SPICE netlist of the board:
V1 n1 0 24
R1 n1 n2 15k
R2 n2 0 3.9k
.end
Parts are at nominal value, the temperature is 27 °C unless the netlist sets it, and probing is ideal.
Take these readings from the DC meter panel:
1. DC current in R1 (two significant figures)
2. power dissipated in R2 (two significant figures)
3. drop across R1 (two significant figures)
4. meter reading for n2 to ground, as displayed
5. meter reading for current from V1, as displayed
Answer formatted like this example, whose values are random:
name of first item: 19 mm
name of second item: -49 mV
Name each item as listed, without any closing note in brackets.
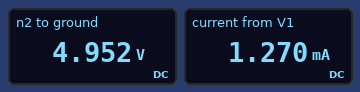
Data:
DC current in R1: 1.3 mA
power dissipated in R2: 6.3 mW
drop across R1: 19 V
meter reading for n2 to ground, as displayed: 4.952 V
meter reading for current from V1, as displayed: 1.270 mA
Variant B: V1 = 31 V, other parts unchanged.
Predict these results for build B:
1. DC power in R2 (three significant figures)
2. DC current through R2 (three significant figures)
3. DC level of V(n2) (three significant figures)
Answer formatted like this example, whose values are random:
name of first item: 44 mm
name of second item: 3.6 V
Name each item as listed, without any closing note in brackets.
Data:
DC power in R2: 10.5 mW
DC current through R2: 1.64 mA
DC level of V(n2): 6.40 V
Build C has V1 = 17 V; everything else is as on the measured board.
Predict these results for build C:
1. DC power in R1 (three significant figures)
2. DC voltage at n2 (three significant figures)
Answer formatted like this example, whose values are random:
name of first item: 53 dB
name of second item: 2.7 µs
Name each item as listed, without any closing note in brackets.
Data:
DC power in R1: 12.1 mW
DC voltage at n2: 3.51 V
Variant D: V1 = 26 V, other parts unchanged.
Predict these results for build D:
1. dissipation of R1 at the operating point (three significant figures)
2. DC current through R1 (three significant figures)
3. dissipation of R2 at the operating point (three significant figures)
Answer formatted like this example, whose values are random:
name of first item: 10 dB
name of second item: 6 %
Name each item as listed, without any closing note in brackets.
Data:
dissipation of R1 at the operating point: 28.4 mW
DC current through R1: 1.38 mA
dissipation of R2 at the operating point: 7.38 mW
